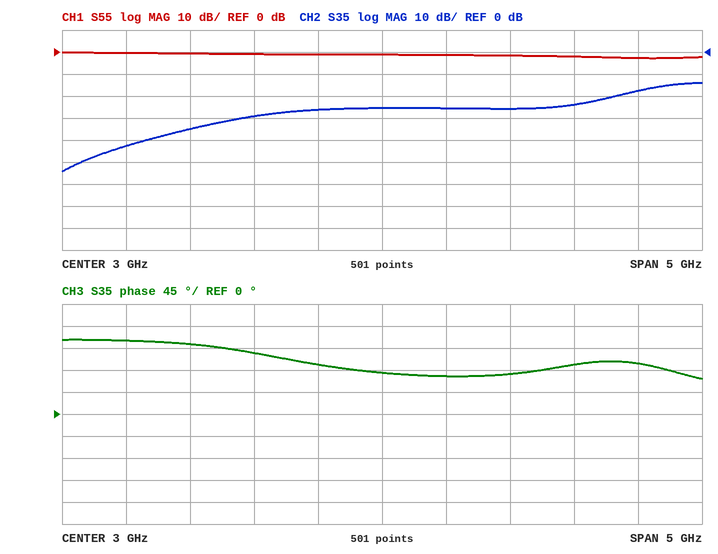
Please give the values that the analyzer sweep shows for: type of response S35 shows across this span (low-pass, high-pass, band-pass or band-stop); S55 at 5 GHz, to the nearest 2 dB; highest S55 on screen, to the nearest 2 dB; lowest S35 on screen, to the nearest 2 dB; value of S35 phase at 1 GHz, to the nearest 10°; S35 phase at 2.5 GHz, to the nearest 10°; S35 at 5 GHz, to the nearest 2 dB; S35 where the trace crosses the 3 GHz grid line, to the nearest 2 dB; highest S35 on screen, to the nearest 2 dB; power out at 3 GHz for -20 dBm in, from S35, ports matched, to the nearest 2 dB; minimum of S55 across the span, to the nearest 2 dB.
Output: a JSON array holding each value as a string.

["high-pass", "-2 dB", "0 dB", "-54 dB", "150°", "100°", "-18 dB", "-26 dB", "-14 dB", "-46 dBm", "-2 dB"]
